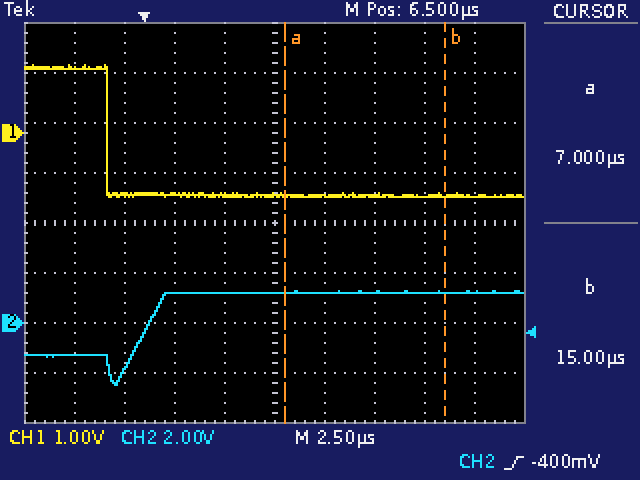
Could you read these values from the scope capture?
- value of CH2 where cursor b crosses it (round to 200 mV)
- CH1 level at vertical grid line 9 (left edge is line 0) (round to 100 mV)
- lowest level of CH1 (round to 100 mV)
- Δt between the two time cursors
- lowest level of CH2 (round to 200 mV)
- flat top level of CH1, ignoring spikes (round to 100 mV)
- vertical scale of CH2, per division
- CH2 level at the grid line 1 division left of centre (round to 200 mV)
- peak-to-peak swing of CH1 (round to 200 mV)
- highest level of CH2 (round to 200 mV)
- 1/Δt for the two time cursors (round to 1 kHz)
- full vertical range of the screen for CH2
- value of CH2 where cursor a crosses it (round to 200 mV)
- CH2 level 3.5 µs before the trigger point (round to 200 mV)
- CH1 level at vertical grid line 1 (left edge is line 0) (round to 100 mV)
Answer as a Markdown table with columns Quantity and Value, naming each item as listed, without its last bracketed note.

| Quantity | Value |
|---|---|
| value of CH2 where cursor b crosses it | 1.2 V |
| CH1 level at vertical grid line 9 (left edge is line 0) | -1.3 V |
| lowest level of CH1 | -1.3 V |
| Δt between the two time cursors | 8.00 µs |
| lowest level of CH2 | -2.4 V |
| flat top level of CH1, ignoring spikes | 1.3 V |
| vertical scale of CH2, per division | 2 V |
| CH2 level at the grid line 1 division left of centre | 1.2 V |
| peak-to-peak swing of CH1 | 2.6 V |
| highest level of CH2 | 1.2 V |
| 1/Δt for the two time cursors | 125 kHz |
| full vertical range of the screen for CH2 | 16 V |
| value of CH2 where cursor a crosses it | 1.2 V |
| CH2 level 3.5 µs before the trigger point | -1.2 V |
| CH1 level at vertical grid line 1 (left edge is line 0) | 1.3 V |
